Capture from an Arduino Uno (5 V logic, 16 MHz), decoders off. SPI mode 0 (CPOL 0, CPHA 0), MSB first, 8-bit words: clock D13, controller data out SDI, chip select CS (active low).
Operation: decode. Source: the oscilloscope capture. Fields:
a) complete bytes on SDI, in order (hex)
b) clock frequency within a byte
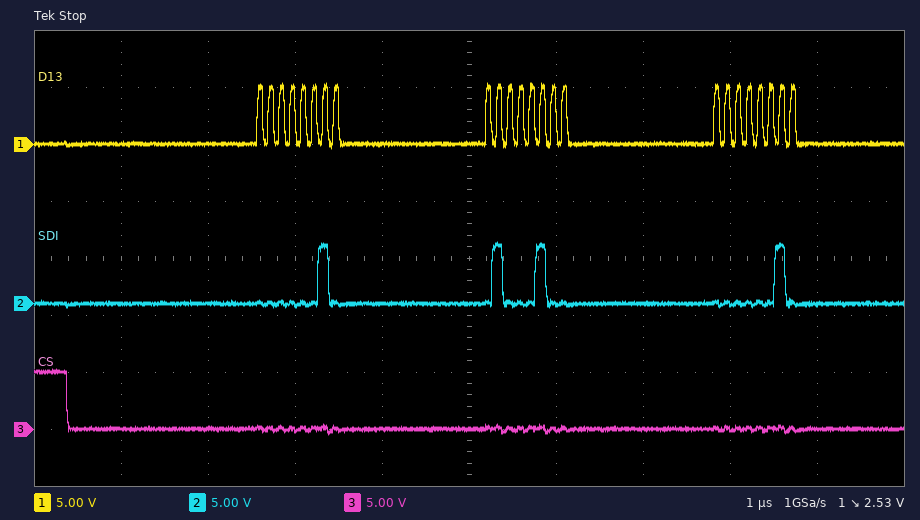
02 44 02
8 MHz
